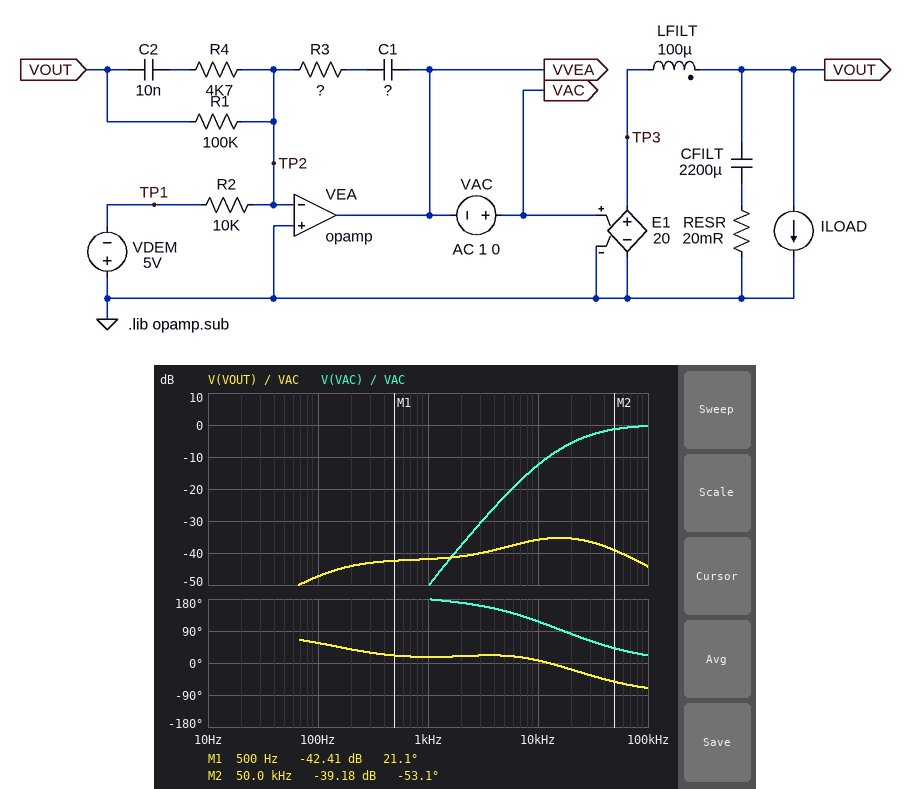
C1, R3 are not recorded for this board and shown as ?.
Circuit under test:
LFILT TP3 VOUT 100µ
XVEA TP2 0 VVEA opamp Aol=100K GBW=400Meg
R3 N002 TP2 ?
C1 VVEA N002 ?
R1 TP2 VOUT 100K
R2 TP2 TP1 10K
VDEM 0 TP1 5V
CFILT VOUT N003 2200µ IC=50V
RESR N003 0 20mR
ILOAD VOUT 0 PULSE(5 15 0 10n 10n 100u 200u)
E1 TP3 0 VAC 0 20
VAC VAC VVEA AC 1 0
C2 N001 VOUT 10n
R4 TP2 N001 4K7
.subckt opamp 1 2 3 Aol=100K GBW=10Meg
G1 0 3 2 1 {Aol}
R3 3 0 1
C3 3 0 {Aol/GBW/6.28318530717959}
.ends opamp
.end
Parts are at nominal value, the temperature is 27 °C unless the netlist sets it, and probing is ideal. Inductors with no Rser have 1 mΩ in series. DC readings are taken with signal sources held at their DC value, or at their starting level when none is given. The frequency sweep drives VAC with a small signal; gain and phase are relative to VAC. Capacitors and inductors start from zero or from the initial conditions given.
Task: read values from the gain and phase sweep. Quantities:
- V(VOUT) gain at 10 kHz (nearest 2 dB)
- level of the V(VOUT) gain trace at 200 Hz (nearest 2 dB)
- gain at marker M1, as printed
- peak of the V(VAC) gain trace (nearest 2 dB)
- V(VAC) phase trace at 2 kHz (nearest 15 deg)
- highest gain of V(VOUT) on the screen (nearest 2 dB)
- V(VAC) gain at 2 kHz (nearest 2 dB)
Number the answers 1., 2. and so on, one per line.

1. -36 dB
2. -44 dB
3. -42.41 dB
4. 0 dB
5. 165 deg
6. -36 dB
7. -38 dB
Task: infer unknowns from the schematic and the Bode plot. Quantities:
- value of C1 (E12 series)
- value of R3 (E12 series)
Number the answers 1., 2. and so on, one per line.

1. 82 pF
2. 270 kΩ
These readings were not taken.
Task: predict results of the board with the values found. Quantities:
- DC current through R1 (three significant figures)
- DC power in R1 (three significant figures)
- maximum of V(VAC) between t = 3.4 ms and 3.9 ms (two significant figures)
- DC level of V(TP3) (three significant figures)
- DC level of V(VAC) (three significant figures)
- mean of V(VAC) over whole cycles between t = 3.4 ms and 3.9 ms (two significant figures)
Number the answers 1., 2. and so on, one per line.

1. 500 µA
2. 25.0 mW
3. 14 V
4. 50.0 V
5. 2.50 V
6. 2.4 V
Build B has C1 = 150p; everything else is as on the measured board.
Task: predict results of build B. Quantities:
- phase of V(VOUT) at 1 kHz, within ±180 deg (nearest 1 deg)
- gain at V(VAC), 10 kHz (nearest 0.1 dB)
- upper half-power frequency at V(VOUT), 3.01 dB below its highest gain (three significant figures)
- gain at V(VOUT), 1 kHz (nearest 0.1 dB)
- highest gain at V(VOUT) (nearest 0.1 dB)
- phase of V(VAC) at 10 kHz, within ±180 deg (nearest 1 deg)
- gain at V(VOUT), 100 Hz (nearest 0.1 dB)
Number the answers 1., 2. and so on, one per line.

1. 11 deg
2. -11.7 dB
3. 39.0 kHz
4. -36.8 dB
5. -35.1 dB
6. 100 deg
7. -42.1 dB
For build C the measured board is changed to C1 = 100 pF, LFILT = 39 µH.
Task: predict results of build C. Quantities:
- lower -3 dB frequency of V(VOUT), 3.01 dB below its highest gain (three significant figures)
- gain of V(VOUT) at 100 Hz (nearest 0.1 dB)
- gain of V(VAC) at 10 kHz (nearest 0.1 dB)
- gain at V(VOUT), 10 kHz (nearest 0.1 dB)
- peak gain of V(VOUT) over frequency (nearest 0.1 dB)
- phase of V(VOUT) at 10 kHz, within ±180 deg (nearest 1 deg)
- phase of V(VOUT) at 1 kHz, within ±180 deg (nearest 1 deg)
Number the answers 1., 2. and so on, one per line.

1. 3.45 kHz
2. -45.6 dB
3. -20.8 dB
4. -36.0 dB
5. -35.4 dB
6. 8 deg
7. 15 deg
